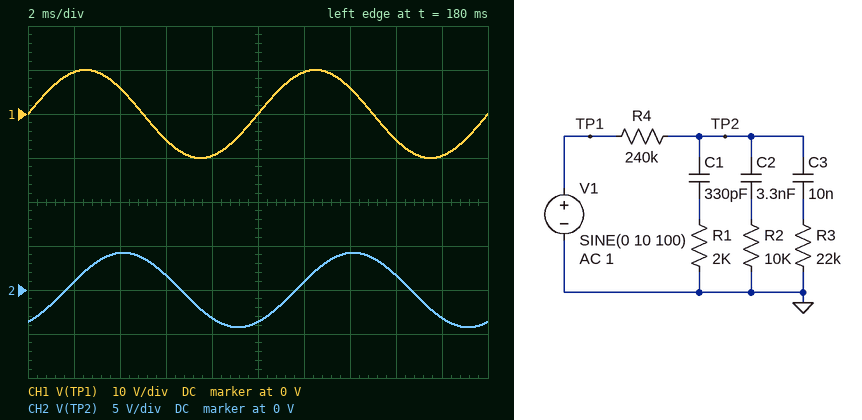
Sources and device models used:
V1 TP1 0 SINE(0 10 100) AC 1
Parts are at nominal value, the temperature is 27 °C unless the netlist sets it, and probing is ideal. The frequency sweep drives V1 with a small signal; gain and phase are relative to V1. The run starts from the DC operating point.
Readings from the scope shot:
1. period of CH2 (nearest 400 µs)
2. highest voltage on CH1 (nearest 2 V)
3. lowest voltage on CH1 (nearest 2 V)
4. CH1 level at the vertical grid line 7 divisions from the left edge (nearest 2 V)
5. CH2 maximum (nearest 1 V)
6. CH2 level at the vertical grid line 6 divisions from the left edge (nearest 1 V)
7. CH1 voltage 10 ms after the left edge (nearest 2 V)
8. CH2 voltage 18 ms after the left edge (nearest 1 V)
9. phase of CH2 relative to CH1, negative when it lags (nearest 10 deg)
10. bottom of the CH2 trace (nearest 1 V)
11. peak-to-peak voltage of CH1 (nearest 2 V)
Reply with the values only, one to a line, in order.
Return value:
10.0 ms
10 V
-10 V
6 V
4 V
1 V
0 V
-3 V
-60 deg
-4 V
20 V
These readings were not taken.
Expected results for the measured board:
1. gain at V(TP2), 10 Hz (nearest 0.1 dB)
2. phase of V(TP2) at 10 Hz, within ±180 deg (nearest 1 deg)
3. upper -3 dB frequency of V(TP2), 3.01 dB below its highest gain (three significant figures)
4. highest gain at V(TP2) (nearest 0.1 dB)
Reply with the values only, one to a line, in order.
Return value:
-0.2 dB
-12 deg
46.4 Hz
0 dB
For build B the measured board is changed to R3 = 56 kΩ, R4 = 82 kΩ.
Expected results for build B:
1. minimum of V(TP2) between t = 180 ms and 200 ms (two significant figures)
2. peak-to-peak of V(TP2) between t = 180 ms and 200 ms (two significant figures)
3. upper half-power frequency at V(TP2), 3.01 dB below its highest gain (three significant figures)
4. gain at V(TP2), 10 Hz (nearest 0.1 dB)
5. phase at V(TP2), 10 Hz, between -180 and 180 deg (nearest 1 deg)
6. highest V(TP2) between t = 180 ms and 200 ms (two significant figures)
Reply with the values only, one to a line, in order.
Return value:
-7.5 V
15 V
116 Hz
0 dB
-4 deg
7.5 V
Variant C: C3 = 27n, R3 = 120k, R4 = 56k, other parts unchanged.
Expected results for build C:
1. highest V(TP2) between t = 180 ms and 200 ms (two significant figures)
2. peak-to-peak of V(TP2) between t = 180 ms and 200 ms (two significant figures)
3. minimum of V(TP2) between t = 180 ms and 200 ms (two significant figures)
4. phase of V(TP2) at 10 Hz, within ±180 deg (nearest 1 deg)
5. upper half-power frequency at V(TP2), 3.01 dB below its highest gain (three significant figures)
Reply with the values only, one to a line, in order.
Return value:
7.1 V
14 V
-7.1 V
-6 deg
101 Hz
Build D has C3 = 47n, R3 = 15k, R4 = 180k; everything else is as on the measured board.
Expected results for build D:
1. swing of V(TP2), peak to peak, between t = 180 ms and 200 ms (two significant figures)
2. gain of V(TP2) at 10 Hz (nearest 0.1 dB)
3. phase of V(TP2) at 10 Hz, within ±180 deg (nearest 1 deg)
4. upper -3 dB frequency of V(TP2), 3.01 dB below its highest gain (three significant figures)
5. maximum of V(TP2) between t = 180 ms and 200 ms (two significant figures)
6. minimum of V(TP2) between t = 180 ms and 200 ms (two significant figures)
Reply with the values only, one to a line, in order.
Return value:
3.5 V
-1.4 dB
-29 deg
16.4 Hz
1.8 V
-1.8 V
